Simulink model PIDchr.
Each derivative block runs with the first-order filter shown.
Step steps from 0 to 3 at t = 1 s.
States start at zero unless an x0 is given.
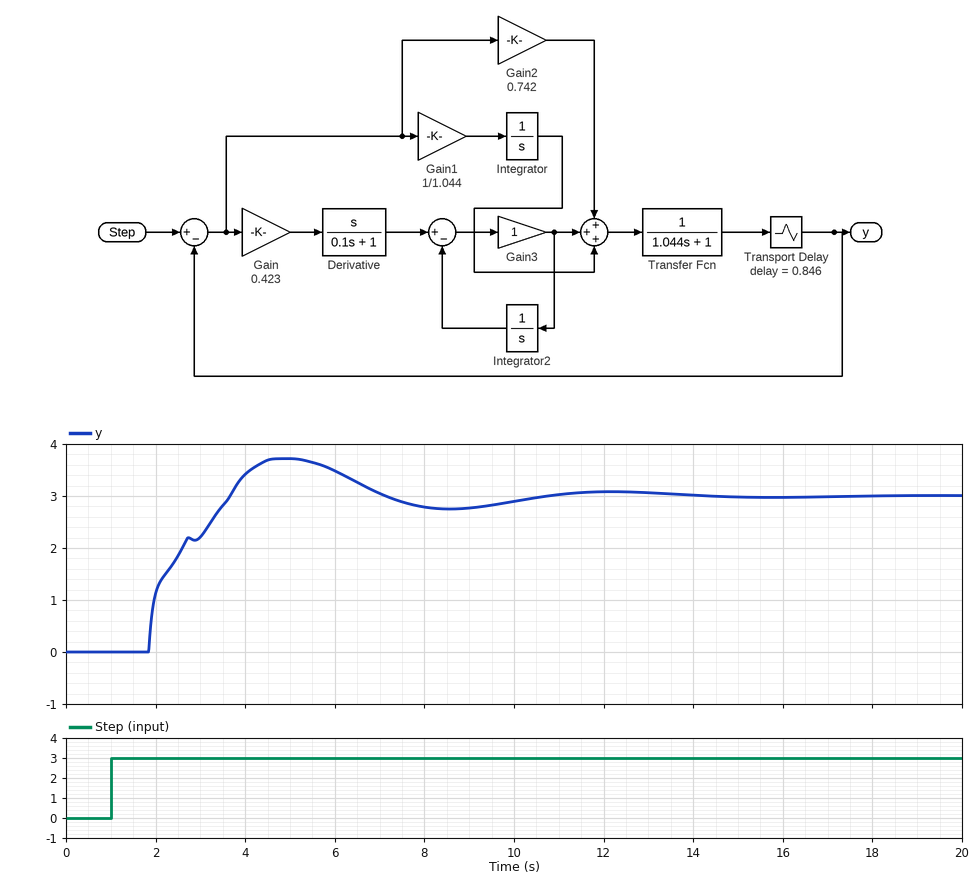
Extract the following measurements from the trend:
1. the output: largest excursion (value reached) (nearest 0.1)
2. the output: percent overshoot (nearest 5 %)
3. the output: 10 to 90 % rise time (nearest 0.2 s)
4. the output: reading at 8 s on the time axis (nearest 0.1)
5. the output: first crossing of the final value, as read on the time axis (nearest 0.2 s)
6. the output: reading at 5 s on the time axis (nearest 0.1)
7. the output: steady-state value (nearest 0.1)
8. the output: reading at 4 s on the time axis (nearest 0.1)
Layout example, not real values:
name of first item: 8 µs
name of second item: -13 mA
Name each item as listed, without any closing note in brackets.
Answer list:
the output: largest excursion (value reached): 3.7
the output: percent overshoot: 25 %
the output: 10 to 90 % rise time: 1.6 s
the output: reading at 8 s on the time axis: 2.8
the output: first crossing of the final value, as read on the time axis: 3.6 s
the output: reading at 5 s on the time axis: 3.7
the output: steady-state value: 3.0
the output: reading at 4 s on the time axis: 3.4
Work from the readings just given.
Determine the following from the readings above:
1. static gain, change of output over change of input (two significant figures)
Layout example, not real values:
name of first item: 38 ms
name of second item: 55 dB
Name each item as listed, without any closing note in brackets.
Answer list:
static gain, change of output over change of input: 1.0
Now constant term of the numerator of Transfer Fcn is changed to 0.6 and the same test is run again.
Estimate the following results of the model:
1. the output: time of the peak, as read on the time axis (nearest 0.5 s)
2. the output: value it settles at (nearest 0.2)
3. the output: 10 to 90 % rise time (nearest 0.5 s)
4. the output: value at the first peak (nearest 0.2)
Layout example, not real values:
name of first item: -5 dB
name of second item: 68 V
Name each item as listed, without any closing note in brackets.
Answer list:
the output: time of the peak, as read on the time axis: 6.5 s
the output: value it settles at: 3.0
the output: 10 to 90 % rise time: 2.5 s
the output: value at the first peak: 3.4
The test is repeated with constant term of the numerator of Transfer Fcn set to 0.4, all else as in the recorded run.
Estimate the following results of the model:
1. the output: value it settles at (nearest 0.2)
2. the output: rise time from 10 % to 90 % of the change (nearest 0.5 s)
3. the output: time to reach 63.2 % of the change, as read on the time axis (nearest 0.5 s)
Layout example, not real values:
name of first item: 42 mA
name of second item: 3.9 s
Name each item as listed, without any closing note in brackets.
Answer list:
the output: value it settles at: 3.0
the output: rise time from 10 % to 90 % of the change: 3.5 s
the output: time to reach 63.2 % of the change, as read on the time axis: 4.0 s
